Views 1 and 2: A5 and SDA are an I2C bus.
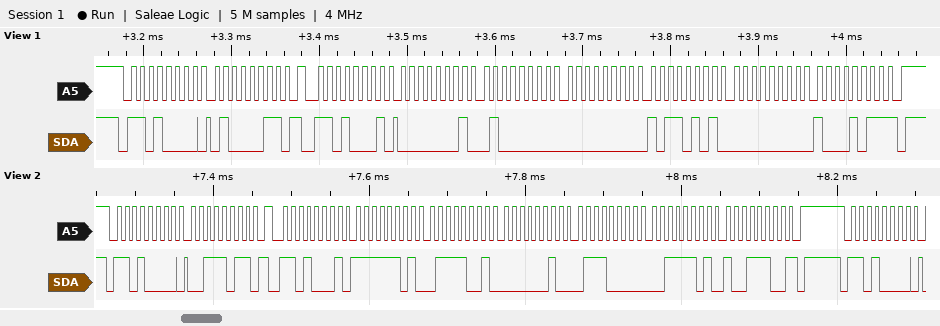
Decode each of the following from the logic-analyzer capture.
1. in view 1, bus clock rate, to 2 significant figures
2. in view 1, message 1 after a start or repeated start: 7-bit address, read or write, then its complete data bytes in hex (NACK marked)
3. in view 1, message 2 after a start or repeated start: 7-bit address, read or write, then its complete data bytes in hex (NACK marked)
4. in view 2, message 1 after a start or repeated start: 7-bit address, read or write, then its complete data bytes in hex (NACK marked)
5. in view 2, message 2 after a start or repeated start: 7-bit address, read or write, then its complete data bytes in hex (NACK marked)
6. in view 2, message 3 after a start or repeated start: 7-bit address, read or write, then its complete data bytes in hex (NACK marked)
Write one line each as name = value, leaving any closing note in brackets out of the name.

in view 1, bus clock rate, to 2 significant figures = 100 kHz
in view 1, message 1 after a start or repeated start: 7-bit address, read or write, then its complete data bytes in hex = 0x68 write: 43
in view 1, message 2 after a start or repeated start: 7-bit address, read or write, then its complete data bytes in hex = 0x68 read: 01 40 00 B5 00 8B NACK
in view 2, message 1 after a start or repeated start: 7-bit address, read or write, then its complete data bytes in hex = 0x68 write: 3B
in view 2, message 2 after a start or repeated start: 7-bit address, read or write, then its complete data bytes in hex = 0x68 read: FD 79 02 70 3D 9C NACK
in view 2, message 3 after a start or repeated start: 7-bit address, read or write, then its complete data bytes in hex = 0x68 write
